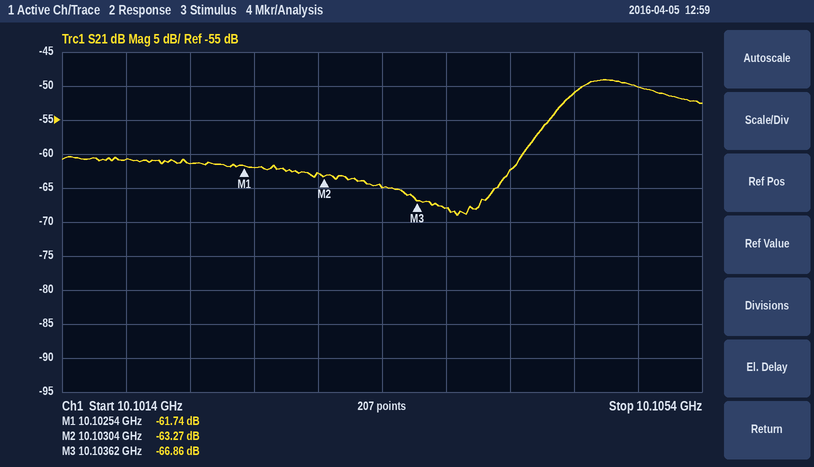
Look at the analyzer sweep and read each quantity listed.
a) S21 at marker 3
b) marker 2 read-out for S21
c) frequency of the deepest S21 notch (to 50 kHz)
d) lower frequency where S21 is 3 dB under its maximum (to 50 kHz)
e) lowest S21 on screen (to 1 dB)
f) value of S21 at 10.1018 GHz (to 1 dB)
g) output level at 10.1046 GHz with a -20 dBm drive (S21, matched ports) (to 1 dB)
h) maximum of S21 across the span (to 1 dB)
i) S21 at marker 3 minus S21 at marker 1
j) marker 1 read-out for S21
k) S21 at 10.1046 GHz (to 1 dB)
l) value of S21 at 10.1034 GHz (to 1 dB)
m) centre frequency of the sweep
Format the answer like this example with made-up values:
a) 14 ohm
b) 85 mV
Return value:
a) -66.86 dB
b) -63.27 dB
c) 10.10385 GHz
d) 10.10455 GHz
e) -69 dB
f) -61 dB
g) -71 dBm
h) -49 dB
i) -5.12 dB
j) -61.74 dB
k) -51 dB
l) -65 dB
m) 10.1034 GHz
